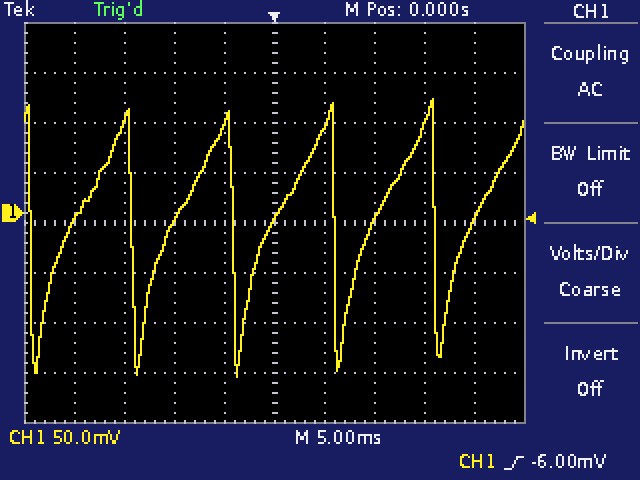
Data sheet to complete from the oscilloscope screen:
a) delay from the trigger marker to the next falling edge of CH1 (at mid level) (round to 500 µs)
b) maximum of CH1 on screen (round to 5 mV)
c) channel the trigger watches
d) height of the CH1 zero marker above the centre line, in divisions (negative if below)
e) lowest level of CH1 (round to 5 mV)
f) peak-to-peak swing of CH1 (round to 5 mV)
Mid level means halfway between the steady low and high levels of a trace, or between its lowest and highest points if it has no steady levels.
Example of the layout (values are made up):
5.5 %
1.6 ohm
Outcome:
6.0 ms
115 mV
CH1
+0.2 div
-165 mV
280 mV
